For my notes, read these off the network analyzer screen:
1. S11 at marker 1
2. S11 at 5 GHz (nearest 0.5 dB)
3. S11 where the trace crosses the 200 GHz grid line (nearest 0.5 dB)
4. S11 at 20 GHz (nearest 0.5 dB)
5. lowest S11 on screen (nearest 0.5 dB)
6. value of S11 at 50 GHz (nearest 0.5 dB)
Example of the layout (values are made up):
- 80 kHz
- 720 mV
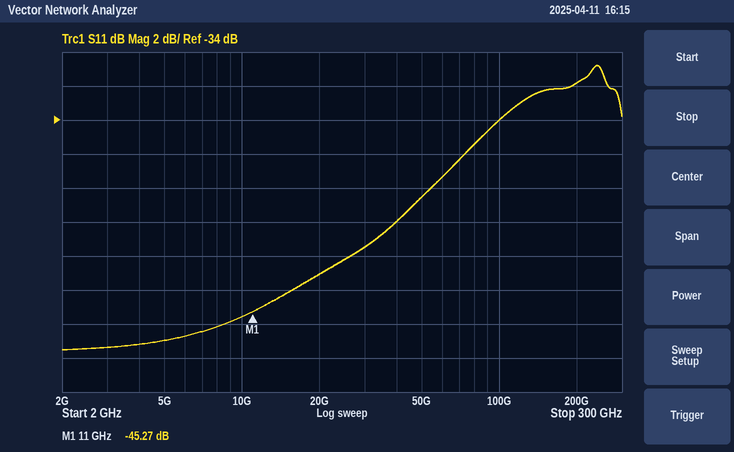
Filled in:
- -45.27 dB
- -47.0 dB
- -32.0 dB
- -43.0 dB
- -47.5 dB
- -38.5 dB
